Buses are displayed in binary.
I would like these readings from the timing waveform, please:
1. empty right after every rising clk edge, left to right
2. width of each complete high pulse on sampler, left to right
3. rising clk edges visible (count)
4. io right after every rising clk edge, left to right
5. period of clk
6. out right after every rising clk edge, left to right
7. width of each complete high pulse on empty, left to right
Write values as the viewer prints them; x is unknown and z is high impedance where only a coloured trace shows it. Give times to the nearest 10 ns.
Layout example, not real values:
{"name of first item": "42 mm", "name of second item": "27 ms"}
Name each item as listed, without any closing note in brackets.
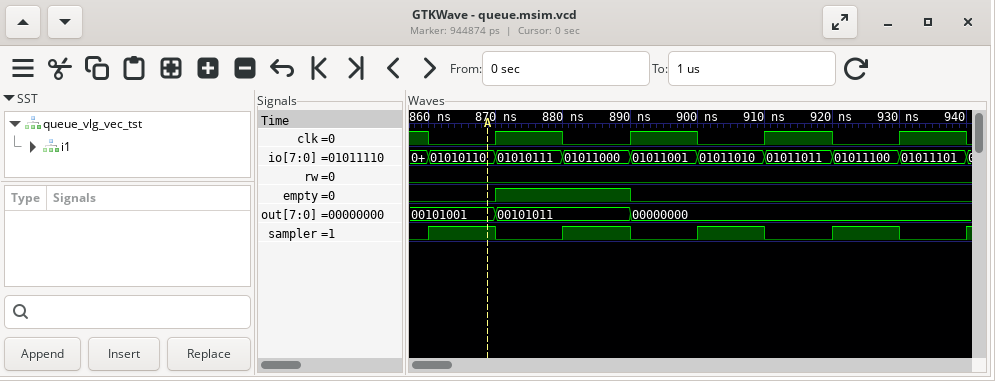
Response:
{"empty right after every rising clk edge, left to right": "1 0 0 0", "width of each complete high pulse on sampler, left to right": "10 ns, 10 ns, 10 ns, 10 ns", "rising clk edges visible": "4", "io right after every rising clk edge, left to right": "01010111, 01011001, 01011011, 01011101", "period of clk": "20 ns", "out right after every rising clk edge, left to right": "00101011, 00000000, 00000000, 00000000", "width of each complete high pulse on empty, left to right": "20 ns"}
